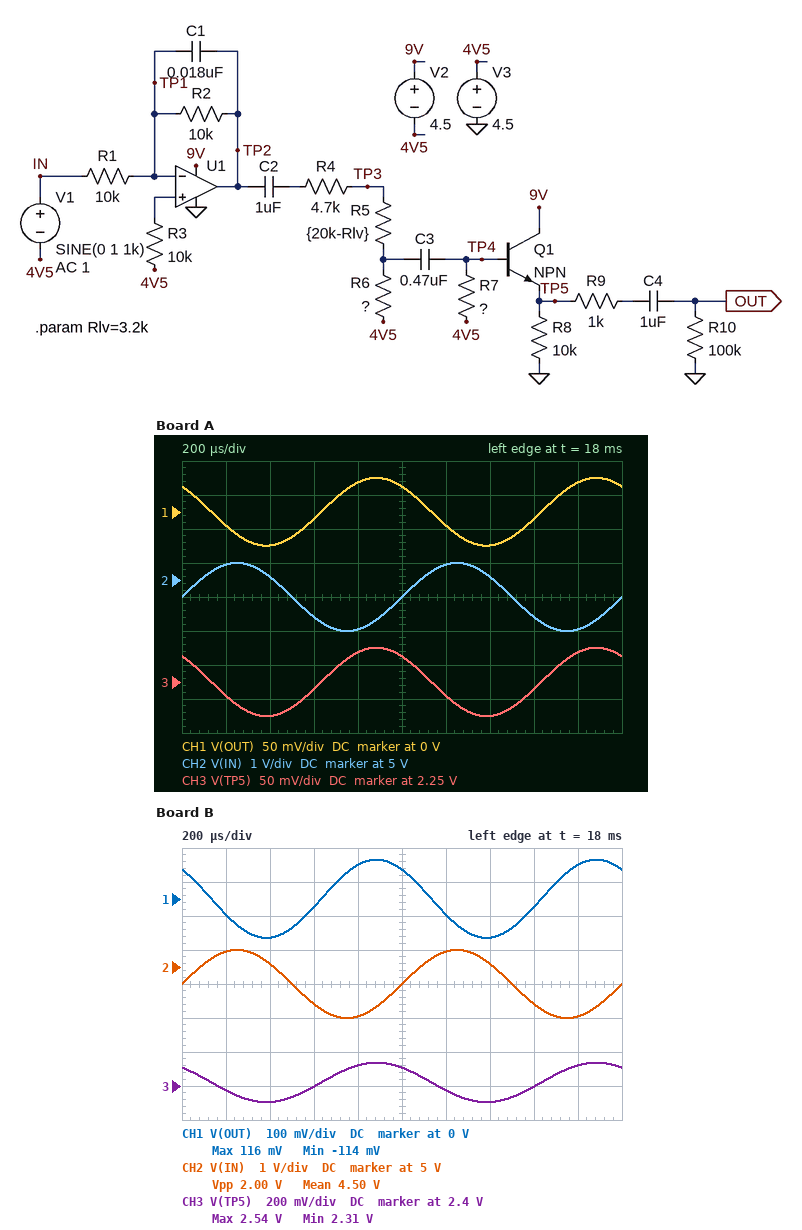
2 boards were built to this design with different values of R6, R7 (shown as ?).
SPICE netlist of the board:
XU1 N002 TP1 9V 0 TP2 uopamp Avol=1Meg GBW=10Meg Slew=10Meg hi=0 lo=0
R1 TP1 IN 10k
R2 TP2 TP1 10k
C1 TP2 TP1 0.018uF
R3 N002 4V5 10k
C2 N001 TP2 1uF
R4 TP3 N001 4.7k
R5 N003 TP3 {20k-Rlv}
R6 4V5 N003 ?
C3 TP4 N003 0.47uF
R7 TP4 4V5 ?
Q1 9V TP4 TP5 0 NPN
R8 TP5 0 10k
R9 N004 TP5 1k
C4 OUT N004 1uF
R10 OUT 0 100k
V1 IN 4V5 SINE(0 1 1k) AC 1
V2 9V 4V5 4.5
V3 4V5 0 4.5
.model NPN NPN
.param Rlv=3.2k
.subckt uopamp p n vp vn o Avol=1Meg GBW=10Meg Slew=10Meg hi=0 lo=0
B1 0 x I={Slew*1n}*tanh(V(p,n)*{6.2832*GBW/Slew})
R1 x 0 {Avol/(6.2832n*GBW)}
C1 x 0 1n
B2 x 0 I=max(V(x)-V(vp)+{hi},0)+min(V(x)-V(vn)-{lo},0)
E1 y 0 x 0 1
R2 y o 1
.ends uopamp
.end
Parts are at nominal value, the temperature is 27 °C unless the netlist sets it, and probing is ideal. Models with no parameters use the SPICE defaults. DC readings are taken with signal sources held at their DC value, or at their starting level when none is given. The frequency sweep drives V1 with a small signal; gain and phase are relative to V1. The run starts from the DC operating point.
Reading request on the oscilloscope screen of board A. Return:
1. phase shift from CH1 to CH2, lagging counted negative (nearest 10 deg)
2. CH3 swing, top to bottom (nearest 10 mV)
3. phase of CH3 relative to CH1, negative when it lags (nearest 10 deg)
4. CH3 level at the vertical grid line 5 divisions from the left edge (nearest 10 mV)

-130 deg
100 mV
0 deg
2.29 V
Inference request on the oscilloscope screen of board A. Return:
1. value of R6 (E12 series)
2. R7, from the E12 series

1.8 kΩ
680 kΩ
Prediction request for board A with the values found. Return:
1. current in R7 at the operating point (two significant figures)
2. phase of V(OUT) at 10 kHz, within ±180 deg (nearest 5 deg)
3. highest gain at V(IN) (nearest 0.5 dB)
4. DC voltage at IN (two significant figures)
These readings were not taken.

2.2 µA
95 deg
0 dB
4.5 V
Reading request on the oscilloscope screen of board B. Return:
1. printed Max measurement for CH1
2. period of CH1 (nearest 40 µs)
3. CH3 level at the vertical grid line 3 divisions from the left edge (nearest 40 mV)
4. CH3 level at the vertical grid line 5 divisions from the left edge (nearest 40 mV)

116 mV
1.00 ms
2.40 V
2.52 V
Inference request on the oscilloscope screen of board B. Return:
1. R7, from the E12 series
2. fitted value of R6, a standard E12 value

560 kΩ
4.7 kΩ
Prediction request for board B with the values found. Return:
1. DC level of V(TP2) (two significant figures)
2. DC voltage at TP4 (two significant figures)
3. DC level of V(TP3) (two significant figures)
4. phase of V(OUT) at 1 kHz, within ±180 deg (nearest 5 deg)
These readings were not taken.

4.5 V
3.2 V
4.5 V
130 deg
